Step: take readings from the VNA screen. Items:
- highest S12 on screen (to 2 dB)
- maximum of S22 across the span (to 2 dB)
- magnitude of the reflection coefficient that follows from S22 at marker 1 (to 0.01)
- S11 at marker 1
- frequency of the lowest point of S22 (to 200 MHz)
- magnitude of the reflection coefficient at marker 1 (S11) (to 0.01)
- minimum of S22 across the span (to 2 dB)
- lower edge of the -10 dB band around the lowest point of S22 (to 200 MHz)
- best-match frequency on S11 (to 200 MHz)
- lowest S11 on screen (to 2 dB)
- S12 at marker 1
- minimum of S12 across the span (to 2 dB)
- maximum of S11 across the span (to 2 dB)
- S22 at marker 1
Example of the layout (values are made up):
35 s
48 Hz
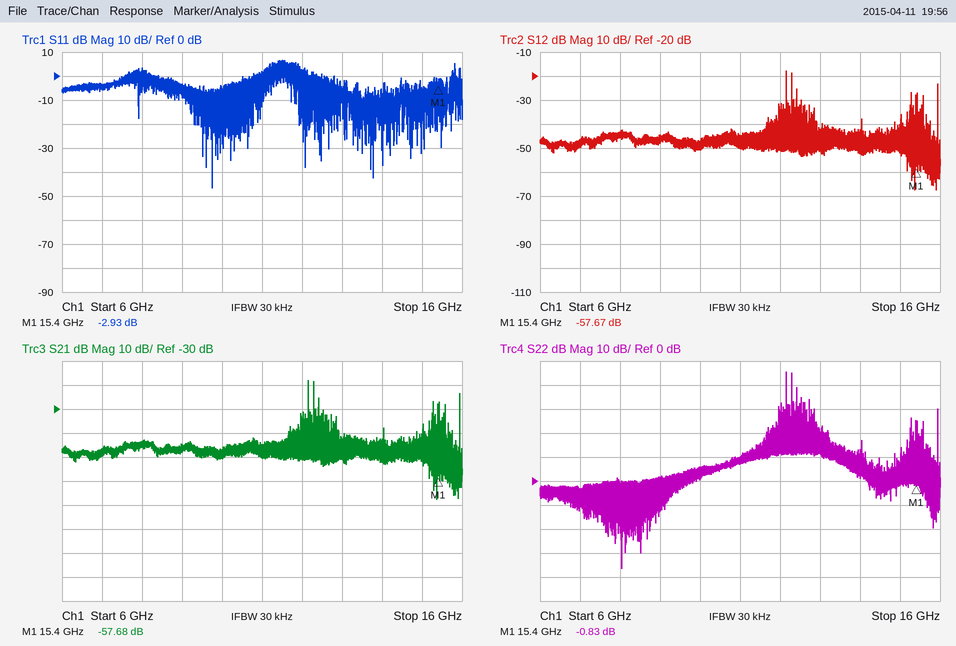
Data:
-18 dB
46 dB
0.91
-2.93 dB
8.0 GHz
0.71
-36 dB
8.0 GHz
9.8 GHz
-46 dB
-57.67 dB
-68 dB
6 dB
-0.83 dB
